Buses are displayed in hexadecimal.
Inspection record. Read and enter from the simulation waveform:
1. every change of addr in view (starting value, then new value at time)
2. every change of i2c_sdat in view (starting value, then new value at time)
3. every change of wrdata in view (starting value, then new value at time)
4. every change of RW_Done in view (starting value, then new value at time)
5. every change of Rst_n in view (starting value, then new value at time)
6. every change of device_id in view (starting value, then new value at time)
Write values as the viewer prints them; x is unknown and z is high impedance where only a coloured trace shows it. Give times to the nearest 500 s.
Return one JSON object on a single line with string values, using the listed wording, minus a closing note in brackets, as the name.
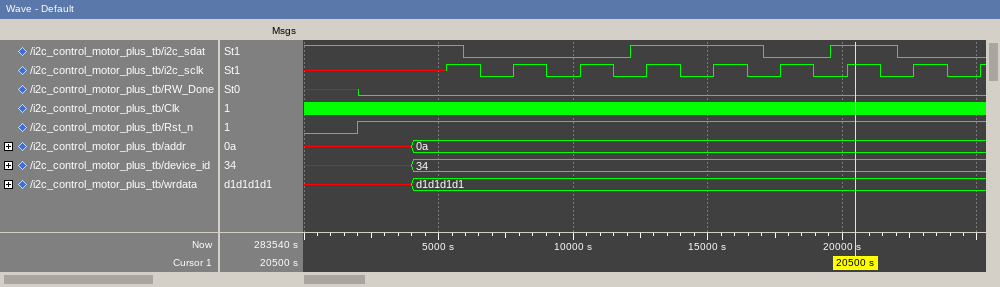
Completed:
{"every change of addr in view": "x, 0a at 4000 s", "every change of i2c_sdat in view": "1, 0 at 6000 s, 1 at 12000 s, 0 at 17000 s, 1 at 19500 s, 0 at 22000 s", "every change of wrdata in view": "x, d1d1d1d1 at 4000 s", "every change of RW_Done in view": "x, 0 at 2000 s", "every change of Rst_n in view": "0, 1 at 2000 s", "every change of device_id in view": "x, 34 at 4000 s"}
